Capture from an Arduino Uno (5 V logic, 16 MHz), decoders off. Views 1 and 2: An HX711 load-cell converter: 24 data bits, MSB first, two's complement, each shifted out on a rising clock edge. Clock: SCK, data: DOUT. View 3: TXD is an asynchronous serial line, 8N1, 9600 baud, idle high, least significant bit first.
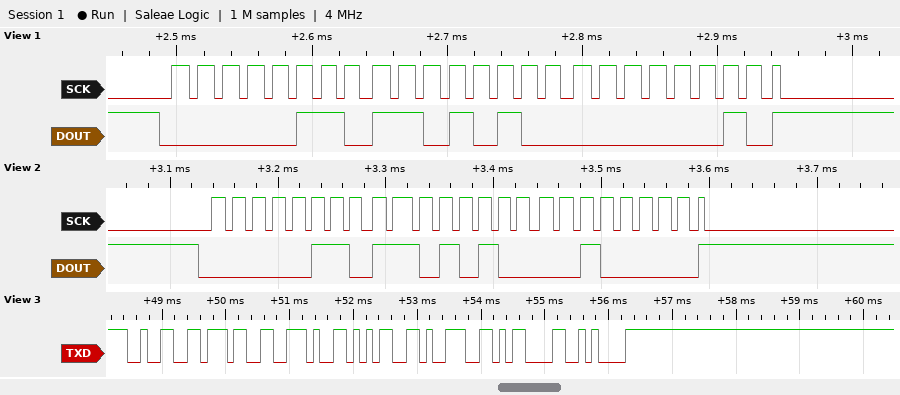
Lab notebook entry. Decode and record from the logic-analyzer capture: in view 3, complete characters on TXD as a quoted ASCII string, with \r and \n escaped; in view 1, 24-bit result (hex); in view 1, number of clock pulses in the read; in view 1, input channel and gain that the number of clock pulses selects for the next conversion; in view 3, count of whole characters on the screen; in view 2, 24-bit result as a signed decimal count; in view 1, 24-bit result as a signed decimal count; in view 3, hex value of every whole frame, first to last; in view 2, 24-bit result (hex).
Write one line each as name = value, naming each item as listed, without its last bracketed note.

in view 3, complete characters on TXD as a quoted ASCII string, with \r and \n escaped = "27.59\r\n"
in view 1, 24-bit result = 0x06D402
in view 1, number of clock pulses in the read = 25
in view 1, input channel and gain that the number of clock pulses selects for the next conversion = channel A, gain 128
in view 3, count of whole characters on the screen = 7
in view 2, 24-bit result as a signed decimal count = 447520
in view 1, 24-bit result as a signed decimal count = 447490
in view 3, hex value of every whole frame, first to last = 32 37 2E 35 39 0D 0A
in view 2, 24-bit result = 0x06D420
